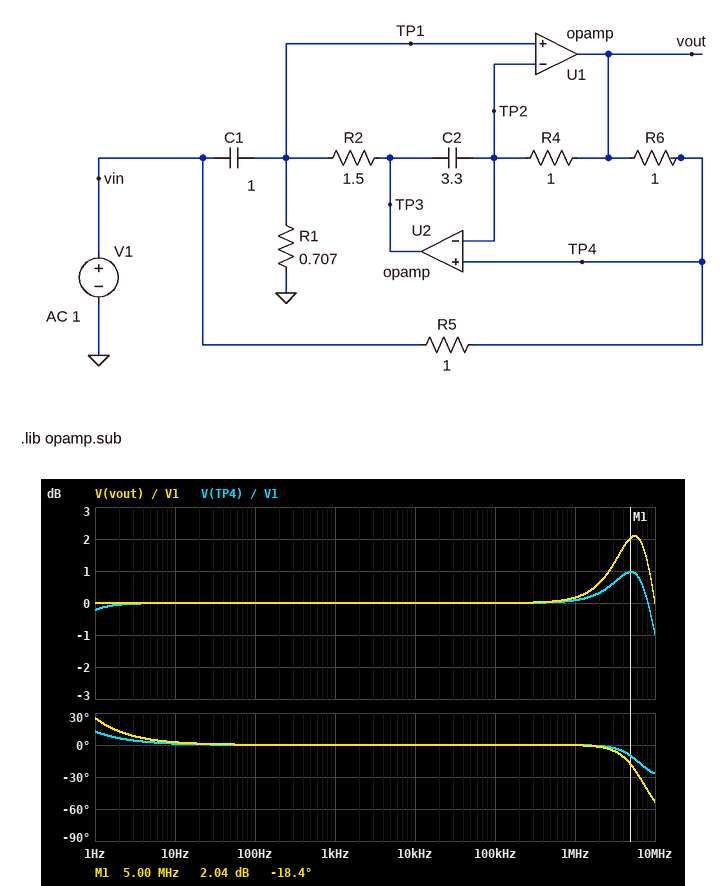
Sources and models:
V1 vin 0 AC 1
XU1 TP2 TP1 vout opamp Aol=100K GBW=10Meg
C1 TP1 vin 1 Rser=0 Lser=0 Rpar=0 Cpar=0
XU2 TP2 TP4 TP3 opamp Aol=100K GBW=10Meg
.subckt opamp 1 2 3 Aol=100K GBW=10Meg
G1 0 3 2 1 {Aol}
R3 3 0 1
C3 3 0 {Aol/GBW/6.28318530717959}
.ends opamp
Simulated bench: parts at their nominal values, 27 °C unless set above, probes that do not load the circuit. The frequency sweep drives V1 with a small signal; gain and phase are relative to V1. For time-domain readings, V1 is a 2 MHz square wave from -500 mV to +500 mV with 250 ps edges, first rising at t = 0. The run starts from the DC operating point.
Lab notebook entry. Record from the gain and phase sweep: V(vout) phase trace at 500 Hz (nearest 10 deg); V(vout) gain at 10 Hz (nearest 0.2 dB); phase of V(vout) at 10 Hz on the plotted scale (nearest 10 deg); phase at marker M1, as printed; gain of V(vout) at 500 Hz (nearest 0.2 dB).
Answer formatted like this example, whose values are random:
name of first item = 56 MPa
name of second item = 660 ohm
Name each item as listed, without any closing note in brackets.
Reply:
V(vout) phase trace at 500 Hz = 0 deg
V(vout) gain at 10 Hz = 0 dB
phase of V(vout) at 10 Hz on the plotted scale = 0 deg
phase at marker M1, as printed = -18.4 deg
gain of V(vout) at 500 Hz = 0 dB
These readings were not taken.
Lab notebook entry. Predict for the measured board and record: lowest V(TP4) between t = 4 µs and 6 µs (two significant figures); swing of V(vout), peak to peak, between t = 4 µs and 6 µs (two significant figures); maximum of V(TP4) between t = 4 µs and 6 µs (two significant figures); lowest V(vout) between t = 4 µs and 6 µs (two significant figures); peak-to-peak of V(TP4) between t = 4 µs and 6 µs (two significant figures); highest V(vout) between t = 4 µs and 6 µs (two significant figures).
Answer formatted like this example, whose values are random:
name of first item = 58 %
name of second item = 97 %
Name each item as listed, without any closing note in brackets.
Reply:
lowest V(TP4) between t = 4 µs and 6 µs = -600 mV
swing of V(vout), peak to peak, between t = 4 µs and 6 µs = 1.4 V
maximum of V(TP4) between t = 4 µs and 6 µs = 600 mV
lowest V(vout) between t = 4 µs and 6 µs = -710 mV
peak-to-peak of V(TP4) between t = 4 µs and 6 µs = 1.2 V
highest V(vout) between t = 4 µs and 6 µs = 710 mV
